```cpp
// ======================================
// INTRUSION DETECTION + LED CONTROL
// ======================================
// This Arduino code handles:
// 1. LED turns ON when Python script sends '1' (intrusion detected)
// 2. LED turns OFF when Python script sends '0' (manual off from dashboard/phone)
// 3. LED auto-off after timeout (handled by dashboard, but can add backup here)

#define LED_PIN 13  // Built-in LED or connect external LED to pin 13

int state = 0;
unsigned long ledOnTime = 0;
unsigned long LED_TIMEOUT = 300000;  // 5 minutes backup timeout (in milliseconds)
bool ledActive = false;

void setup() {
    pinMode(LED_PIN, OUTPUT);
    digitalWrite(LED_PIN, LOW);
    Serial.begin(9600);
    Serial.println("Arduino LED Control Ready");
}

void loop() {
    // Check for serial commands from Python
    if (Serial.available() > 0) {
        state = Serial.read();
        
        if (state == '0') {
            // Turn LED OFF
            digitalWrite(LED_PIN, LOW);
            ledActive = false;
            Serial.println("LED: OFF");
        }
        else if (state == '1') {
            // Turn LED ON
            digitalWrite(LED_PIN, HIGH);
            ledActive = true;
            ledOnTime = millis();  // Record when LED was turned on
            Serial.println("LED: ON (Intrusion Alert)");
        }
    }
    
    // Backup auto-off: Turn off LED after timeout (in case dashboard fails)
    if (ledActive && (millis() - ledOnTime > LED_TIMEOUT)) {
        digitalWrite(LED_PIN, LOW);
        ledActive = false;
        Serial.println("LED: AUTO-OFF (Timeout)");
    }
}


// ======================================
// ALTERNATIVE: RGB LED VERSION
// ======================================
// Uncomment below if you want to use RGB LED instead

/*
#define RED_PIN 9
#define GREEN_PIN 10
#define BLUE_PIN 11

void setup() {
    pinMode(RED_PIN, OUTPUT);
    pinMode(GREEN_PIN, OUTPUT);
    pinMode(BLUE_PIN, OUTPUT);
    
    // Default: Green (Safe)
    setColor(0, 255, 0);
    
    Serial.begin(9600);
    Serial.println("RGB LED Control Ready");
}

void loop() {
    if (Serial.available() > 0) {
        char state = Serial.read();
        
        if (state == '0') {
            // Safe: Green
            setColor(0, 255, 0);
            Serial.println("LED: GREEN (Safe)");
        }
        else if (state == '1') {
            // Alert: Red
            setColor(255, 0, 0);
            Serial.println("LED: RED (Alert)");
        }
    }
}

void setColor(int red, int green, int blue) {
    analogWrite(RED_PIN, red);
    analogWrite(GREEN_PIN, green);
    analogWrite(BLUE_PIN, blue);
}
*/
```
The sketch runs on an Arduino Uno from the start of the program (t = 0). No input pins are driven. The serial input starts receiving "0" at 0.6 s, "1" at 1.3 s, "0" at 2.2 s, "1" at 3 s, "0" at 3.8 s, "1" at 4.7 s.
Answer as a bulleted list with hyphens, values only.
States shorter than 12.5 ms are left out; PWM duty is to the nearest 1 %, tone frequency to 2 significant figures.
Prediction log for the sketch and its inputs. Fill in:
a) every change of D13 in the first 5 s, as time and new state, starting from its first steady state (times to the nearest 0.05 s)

- 0 s low; 1.3 s high; 2.2 s low; 3 s high; 3.8 s low; 4.7 s high
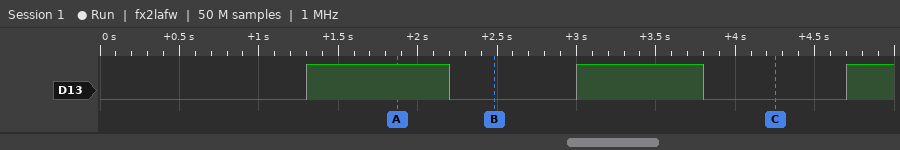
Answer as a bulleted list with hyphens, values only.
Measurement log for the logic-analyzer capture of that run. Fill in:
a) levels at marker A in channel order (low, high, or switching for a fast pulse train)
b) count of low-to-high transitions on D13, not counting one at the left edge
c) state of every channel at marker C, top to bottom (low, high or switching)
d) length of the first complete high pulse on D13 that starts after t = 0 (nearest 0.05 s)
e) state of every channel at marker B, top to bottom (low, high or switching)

- D13 high
- 3
- D13 low
- 0.90 s
- D13 low
